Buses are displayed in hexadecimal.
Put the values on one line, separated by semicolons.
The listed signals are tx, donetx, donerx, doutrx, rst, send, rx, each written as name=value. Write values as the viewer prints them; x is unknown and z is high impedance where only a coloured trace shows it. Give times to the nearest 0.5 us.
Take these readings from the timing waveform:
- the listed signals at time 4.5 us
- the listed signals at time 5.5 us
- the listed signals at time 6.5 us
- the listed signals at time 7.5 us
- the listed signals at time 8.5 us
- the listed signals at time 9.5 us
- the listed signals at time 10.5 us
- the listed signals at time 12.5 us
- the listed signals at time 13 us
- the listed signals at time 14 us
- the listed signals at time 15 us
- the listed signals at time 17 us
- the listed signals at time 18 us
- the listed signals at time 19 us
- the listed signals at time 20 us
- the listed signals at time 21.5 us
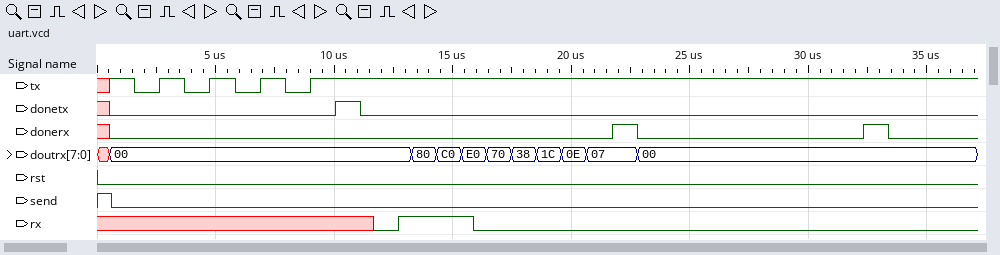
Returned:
tx=0, donetx=0, donerx=0, doutrx=00, rst=0, send=0, rx=x; tx=1, donetx=0, donerx=0, doutrx=00, rst=0, send=0, rx=x; tx=0, donetx=0, donerx=0, doutrx=00, rst=0, send=0, rx=x; tx=1, donetx=0, donerx=0, doutrx=00, rst=0, send=0, rx=x; tx=0, donetx=0, donerx=0, doutrx=00, rst=0, send=0, rx=x; tx=1, donetx=0, donerx=0, doutrx=00, rst=0, send=0, rx=x; tx=1, donetx=1, donerx=0, doutrx=00, rst=0, send=0, rx=x; tx=1, donetx=0, donerx=0, doutrx=00, rst=0, send=0, rx=0; tx=1, donetx=0, donerx=0, doutrx=00, rst=0, send=0, rx=1; tx=1, donetx=0, donerx=0, doutrx=80, rst=0, send=0, rx=1; tx=1, donetx=0, donerx=0, doutrx=C0, rst=0, send=0, rx=1; tx=1, donetx=0, donerx=0, doutrx=70, rst=0, send=0, rx=0; tx=1, donetx=0, donerx=0, doutrx=38, rst=0, send=0, rx=0; tx=1, donetx=0, donerx=0, doutrx=1C, rst=0, send=0, rx=0; tx=1, donetx=0, donerx=0, doutrx=0E, rst=0, send=0, rx=0; tx=1, donetx=0, donerx=0, doutrx=07, rst=0, send=0, rx=0
